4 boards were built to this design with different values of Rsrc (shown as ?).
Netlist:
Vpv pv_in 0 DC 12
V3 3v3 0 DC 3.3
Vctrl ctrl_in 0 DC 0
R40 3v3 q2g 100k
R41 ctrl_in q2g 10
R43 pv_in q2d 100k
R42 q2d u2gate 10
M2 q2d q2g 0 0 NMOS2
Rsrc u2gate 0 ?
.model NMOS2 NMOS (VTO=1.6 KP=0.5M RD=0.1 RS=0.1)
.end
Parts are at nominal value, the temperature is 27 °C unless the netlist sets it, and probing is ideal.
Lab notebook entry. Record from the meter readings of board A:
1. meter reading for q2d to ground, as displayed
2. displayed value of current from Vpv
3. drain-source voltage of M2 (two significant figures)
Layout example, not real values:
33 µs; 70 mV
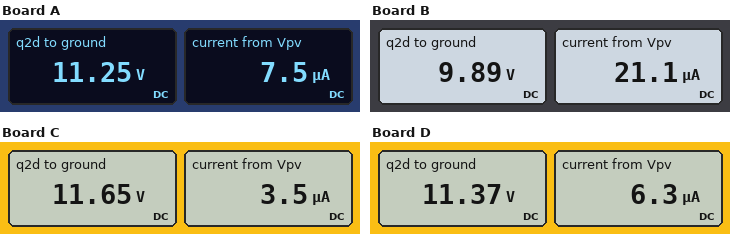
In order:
11.25 V; 7.5 µA; 11 V
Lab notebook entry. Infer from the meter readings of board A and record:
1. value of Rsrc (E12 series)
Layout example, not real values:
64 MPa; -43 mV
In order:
1.5 MΩ
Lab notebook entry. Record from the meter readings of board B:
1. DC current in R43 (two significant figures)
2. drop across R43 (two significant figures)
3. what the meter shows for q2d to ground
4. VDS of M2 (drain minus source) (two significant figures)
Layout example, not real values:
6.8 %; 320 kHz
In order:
21 µA; 2.1 V; 9.89 V; 9.9 V
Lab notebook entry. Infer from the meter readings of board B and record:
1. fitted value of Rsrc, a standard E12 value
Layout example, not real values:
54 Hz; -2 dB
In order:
470 kΩ
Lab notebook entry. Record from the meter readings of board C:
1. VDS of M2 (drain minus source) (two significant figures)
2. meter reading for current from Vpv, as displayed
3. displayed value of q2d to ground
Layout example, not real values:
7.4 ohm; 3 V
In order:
12 V; 3.5 µA; 11.65 V
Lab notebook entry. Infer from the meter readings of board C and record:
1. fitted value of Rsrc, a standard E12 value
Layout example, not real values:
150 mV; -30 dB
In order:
3.3 MΩ
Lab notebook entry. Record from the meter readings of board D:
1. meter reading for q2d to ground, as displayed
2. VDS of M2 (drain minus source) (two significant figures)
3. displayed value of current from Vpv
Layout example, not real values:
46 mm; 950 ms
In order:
11.37 V; 11 V; 6.3 µA
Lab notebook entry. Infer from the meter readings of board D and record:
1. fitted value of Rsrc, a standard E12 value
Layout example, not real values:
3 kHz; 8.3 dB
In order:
1.8 MΩ
